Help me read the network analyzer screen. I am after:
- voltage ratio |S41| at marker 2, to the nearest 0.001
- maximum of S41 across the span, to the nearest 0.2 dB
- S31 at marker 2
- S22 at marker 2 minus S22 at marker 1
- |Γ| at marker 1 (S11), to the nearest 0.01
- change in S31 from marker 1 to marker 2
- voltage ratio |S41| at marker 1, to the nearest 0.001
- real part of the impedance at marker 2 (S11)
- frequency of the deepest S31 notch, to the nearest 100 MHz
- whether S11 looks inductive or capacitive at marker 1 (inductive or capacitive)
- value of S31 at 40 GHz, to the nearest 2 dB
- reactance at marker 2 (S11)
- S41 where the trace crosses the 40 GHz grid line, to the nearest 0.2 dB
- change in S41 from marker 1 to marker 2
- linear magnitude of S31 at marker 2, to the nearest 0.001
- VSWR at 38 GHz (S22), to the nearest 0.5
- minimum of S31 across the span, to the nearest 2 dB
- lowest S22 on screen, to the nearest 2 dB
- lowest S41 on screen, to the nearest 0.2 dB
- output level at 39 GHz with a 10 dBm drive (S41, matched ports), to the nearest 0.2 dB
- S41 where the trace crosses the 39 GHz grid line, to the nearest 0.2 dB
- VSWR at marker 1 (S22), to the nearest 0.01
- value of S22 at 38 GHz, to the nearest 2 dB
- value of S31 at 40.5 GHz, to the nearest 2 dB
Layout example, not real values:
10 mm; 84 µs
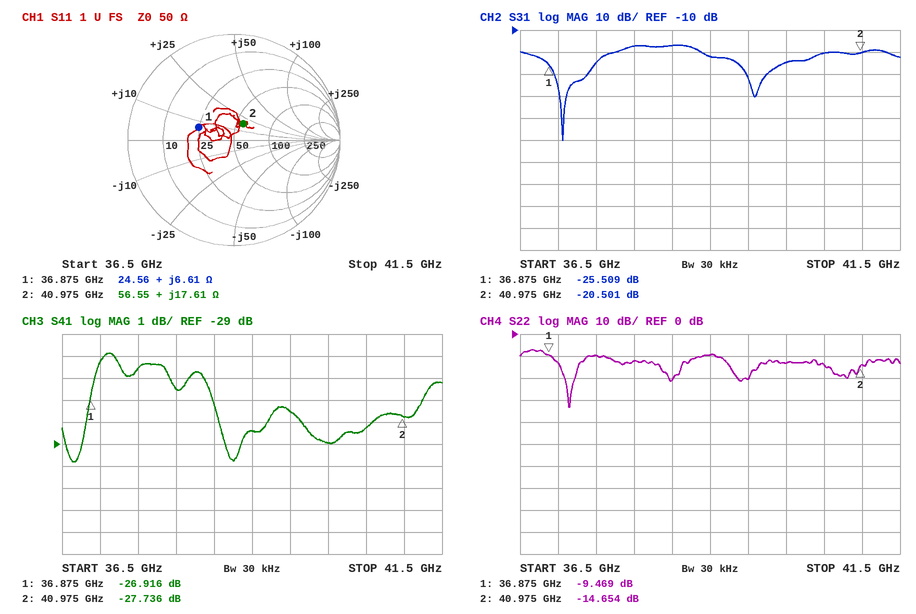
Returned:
0.041; -24.8 dB; -20.501 dB; -5.185 dB; 0.35; 5.008 dB; 0.045; 56.55 Ω; 37.1 GHz; inductive; -24 dB; +17.61 Ω; -29.0 dB; -0.820 dB; 0.094; 1.5; -60 dB; -34 dB; -29.8 dB; -18.4 dBm; -28.4 dB; 2.01; -12 dB; -20 dB
